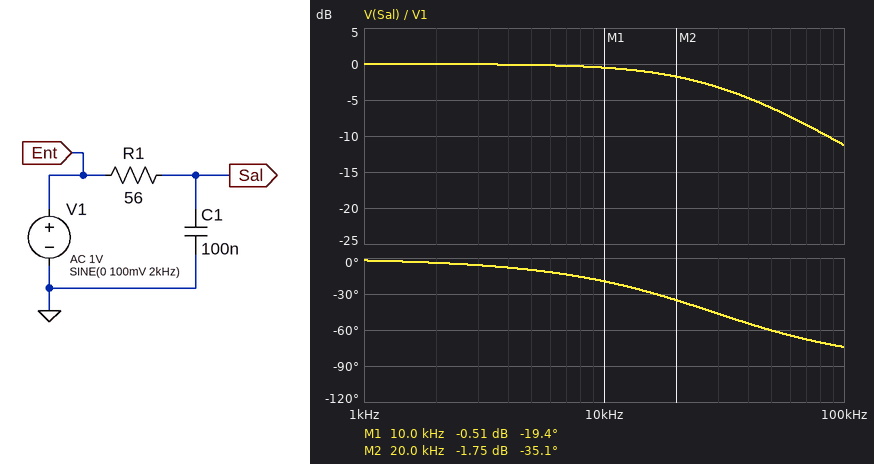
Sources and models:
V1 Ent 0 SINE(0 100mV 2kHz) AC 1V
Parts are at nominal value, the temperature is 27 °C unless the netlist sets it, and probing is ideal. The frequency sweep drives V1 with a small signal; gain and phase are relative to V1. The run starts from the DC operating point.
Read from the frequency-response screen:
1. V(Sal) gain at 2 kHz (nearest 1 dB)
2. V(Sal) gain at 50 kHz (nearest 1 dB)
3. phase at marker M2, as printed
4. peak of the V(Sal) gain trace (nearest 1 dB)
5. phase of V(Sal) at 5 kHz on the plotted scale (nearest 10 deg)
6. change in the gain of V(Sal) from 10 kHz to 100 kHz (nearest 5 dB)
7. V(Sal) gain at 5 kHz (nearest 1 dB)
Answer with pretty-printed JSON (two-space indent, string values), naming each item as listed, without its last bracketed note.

{
  "V(Sal) gain at 2 kHz": "0 dB",
  "V(Sal) gain at 50 kHz": "-6 dB",
  "phase at marker M2, as printed": "-35.1 deg",
  "peak of the V(Sal) gain trace": "0 dB",
  "phase of V(Sal) at 5 kHz on the plotted scale": "-10 deg",
  "change in the gain of V(Sal) from 10 kHz to 100 kHz": "-10 dB",
  "V(Sal) gain at 5 kHz": "0 dB"
}
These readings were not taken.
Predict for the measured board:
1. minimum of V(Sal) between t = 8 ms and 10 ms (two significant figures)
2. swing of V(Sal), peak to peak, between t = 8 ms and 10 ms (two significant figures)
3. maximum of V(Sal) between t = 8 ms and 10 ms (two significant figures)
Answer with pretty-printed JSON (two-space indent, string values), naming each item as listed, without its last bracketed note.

{
  "minimum of V(Sal) between t = 8 ms and 10 ms": "-100 mV",
  "swing of V(Sal), peak to peak, between t = 8 ms and 10 ms": "200 mV",
  "maximum of V(Sal) between t = 8 ms and 10 ms": "100 mV"
}
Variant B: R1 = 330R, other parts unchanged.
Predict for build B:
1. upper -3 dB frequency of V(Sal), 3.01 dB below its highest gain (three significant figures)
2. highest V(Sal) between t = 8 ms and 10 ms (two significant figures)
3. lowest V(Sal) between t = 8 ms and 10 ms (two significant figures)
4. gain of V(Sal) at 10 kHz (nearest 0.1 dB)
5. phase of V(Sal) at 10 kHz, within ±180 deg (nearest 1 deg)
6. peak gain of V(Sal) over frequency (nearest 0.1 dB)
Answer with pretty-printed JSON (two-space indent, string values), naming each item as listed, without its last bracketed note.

{
  "upper -3 dB frequency of V(Sal), 3.01 dB below its highest gain": "4.82 kHz",
  "highest V(Sal) between t = 8 ms and 10 ms": "92 mV",
  "lowest V(Sal) between t = 8 ms and 10 ms": "-92 mV",
  "gain of V(Sal) at 10 kHz": "-7.2 dB",
  "phase of V(Sal) at 10 kHz, within ±180 deg": "-64 deg",
  "peak gain of V(Sal) over frequency": "0 dB"
}
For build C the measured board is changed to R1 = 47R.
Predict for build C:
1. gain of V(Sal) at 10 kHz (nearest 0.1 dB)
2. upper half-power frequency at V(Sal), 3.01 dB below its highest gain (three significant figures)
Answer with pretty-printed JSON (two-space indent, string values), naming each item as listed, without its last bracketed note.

{
  "gain of V(Sal) at 10 kHz": "-0.4 dB",
  "upper half-power frequency at V(Sal), 3.01 dB below its highest gain": "33.9 kHz"
}
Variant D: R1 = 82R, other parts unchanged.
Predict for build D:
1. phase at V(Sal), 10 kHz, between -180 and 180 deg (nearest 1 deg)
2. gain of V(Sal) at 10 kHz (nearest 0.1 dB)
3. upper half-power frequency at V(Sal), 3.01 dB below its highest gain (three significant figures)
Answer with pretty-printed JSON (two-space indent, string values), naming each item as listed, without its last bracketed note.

{
  "phase at V(Sal), 10 kHz, between -180 and 180 deg": "-27 deg",
  "gain of V(Sal) at 10 kHz": "-1.0 dB",
  "upper half-power frequency at V(Sal), 3.01 dB below its highest gain": "19.4 kHz"
}
